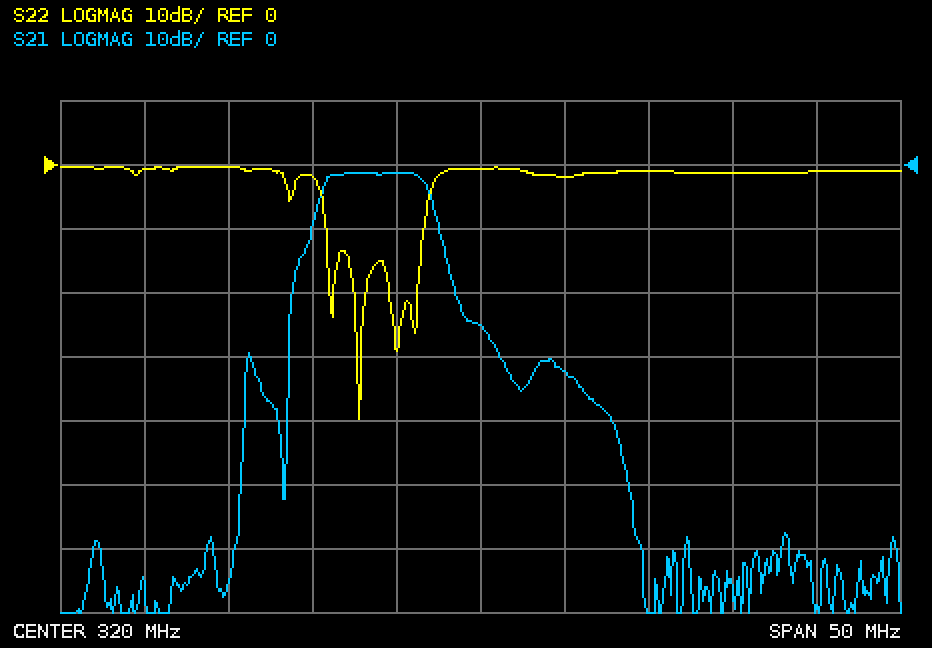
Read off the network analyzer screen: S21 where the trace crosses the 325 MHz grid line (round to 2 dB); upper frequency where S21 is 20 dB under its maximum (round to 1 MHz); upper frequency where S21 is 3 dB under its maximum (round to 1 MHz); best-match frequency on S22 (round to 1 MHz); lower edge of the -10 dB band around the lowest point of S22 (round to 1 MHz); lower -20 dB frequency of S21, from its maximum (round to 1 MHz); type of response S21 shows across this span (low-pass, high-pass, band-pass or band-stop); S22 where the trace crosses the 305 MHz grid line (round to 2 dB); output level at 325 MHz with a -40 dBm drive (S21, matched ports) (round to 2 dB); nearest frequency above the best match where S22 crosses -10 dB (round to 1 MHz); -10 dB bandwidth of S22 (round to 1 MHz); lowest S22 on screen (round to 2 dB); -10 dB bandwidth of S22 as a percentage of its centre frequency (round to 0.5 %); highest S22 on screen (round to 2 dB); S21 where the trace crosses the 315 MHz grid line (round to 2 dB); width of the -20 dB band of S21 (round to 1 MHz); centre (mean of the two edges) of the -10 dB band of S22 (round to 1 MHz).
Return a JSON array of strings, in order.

["-32 dB", "319 MHz", "317 MHz", "313 MHz", "311 MHz", "309 MHz", "band-pass", "0 dB", "-72 dBm", "317 MHz", "6 MHz", "-40 dB", "2.0 %", "0 dB", "-2 dB", "10 MHz", "314 MHz"]
